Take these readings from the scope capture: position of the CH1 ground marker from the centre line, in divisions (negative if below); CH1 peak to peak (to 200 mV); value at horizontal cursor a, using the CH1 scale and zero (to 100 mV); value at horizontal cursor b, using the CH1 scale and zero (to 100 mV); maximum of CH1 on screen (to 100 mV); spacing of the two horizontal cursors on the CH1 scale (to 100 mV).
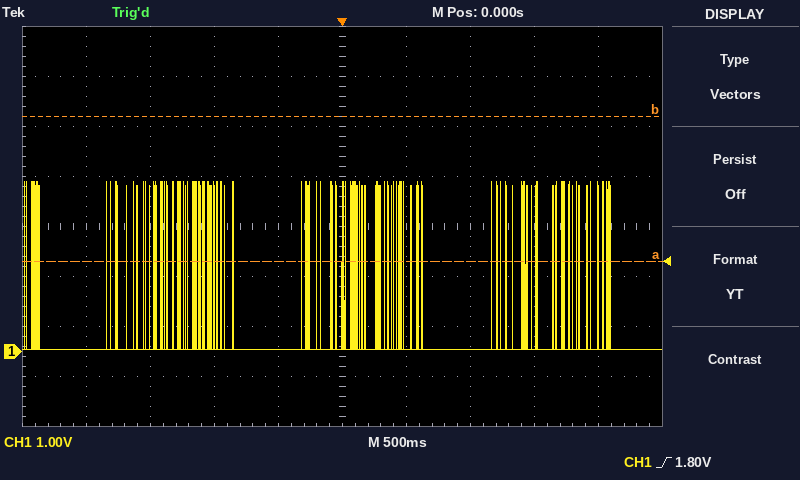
-2.5 div
3.4 V
1.8 V
4.7 V
3.4 V
2.9 V
